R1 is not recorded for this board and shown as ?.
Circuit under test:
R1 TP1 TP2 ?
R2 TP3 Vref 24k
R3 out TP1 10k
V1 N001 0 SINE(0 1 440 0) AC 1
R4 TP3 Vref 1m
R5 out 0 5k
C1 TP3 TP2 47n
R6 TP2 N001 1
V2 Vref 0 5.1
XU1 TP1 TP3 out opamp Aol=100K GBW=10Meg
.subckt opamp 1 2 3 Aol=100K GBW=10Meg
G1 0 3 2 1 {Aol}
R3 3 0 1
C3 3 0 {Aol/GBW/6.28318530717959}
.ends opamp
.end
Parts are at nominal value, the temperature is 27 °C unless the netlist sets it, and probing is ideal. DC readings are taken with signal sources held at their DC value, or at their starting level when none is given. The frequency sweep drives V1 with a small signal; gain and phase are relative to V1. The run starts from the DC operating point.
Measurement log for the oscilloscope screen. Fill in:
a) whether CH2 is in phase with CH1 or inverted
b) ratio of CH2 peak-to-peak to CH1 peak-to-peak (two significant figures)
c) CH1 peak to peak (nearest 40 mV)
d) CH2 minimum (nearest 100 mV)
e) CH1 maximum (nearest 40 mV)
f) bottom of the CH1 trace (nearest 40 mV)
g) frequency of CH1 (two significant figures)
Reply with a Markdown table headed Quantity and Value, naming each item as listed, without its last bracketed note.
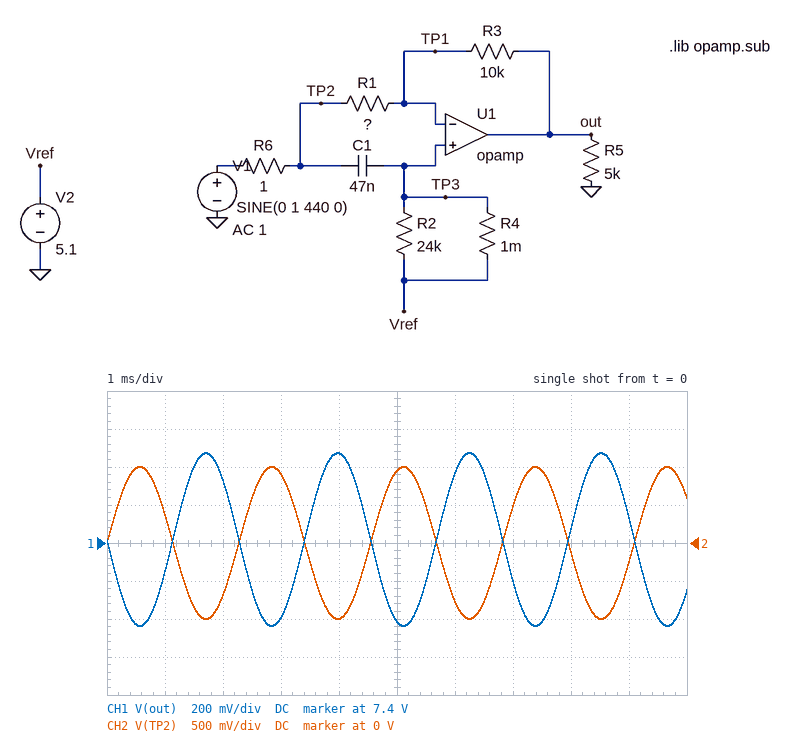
| Quantity | Value |
|---|---|
| whether CH2 is in phase with CH1 or inverted | inverted |
| ratio of CH2 peak-to-peak to CH1 peak-to-peak | 2.2 |
| CH1 peak to peak | 920 mV |
| CH2 minimum | -1.0 V |
| CH1 maximum | 7.88 V |
| bottom of the CH1 trace | 6.96 V |
| frequency of CH1 | 440 Hz |
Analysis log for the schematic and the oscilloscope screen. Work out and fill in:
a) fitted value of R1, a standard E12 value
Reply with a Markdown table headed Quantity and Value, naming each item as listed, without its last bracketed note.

| Quantity | Value |
|---|---|
| fitted value of R1, a standard E12 value | 22 kΩ |
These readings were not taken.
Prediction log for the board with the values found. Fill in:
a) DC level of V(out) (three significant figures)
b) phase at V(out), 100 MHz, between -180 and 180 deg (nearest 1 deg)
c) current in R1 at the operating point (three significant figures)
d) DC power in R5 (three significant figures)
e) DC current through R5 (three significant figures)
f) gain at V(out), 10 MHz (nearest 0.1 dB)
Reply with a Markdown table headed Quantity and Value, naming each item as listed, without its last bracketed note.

| Quantity | Value |
|---|---|
| DC level of V(out) | 7.42 V |
| phase at V(out), 100 MHz, between -180 and 180 deg | 2 deg |
| current in R1 at the operating point | 232 µA |
| DC power in R5 | 11.0 mW |
| DC current through R5 | 1.48 mA |
| gain at V(out), 10 MHz | -21.7 dB |
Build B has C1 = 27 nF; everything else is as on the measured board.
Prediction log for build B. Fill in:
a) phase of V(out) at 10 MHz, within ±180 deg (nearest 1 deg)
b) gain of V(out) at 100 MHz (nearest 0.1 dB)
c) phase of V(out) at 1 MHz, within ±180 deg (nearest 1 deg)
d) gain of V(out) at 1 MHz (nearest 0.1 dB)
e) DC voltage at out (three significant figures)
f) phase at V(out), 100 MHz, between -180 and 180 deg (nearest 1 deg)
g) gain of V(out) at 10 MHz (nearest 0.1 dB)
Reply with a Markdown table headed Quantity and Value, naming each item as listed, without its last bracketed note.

| Quantity | Value |
|---|---|
| phase of V(out) at 10 MHz, within ±180 deg | 65 deg |
| gain of V(out) at 100 MHz | -54.7 dB |
| phase of V(out) at 1 MHz, within ±180 deg | 162 deg |
| gain of V(out) at 1 MHz | -7.1 dB |
| DC voltage at out | 7.42 V |
| phase at V(out), 100 MHz, between -180 and 180 deg | 5 deg |
| gain of V(out) at 10 MHz | -17.7 dB |
